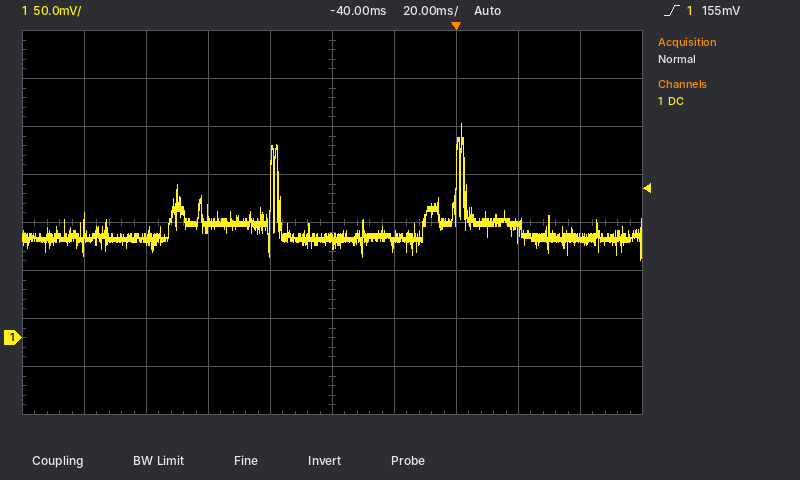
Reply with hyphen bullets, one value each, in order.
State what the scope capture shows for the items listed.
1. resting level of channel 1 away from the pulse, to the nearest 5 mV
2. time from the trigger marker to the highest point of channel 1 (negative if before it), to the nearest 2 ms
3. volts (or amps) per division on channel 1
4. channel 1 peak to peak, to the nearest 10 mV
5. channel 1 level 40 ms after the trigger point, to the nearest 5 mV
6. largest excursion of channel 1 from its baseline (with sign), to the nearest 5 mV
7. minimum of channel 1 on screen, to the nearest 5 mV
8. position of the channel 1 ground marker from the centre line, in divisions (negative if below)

- 105 mV
- +2 ms
- 50 mV
- 140 mV
- 105 mV
- +120 mV
- 80 mV
- -2.4 div
